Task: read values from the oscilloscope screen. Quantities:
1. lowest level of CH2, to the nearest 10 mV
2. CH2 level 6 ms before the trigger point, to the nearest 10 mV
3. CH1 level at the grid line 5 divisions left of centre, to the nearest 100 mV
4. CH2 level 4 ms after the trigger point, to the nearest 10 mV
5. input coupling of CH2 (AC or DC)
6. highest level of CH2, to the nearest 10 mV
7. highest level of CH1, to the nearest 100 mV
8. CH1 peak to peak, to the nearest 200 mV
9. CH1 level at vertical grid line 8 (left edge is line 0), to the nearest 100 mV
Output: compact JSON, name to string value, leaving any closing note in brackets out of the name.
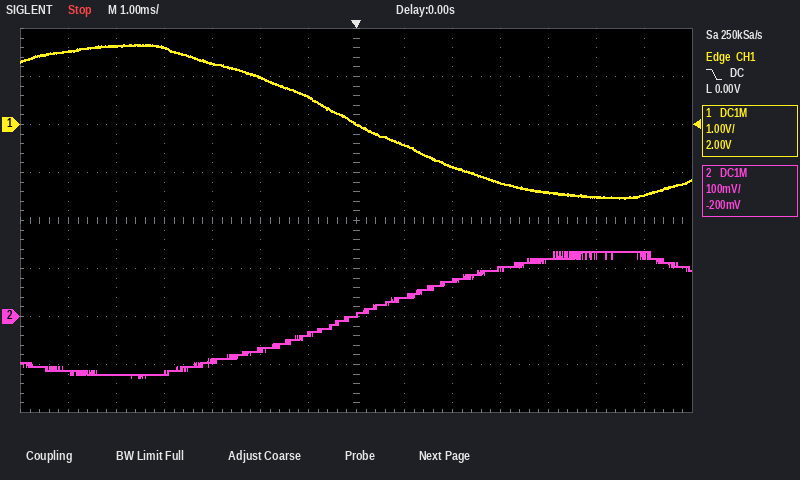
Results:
{"lowest level of CH2, to the nearest 10 mV": "-130 mV", "CH2 level 6 ms before the trigger point, to the nearest 10 mV": "-110 mV", "CH1 level at the grid line 5 divisions left of centre, to the nearest 100 mV": "1.6 V", "CH2 level 4 ms after the trigger point, to the nearest 10 mV": "120 mV", "input coupling of CH2": "DC", "highest level of CH2, to the nearest 10 mV": "140 mV", "highest level of CH1, to the nearest 100 mV": "1.7 V", "CH1 peak to peak, to the nearest 200 mV": "3.2 V", "CH1 level at vertical grid line 8 (left edge is line 0), to the nearest 100 mV": "-400 mV"}
